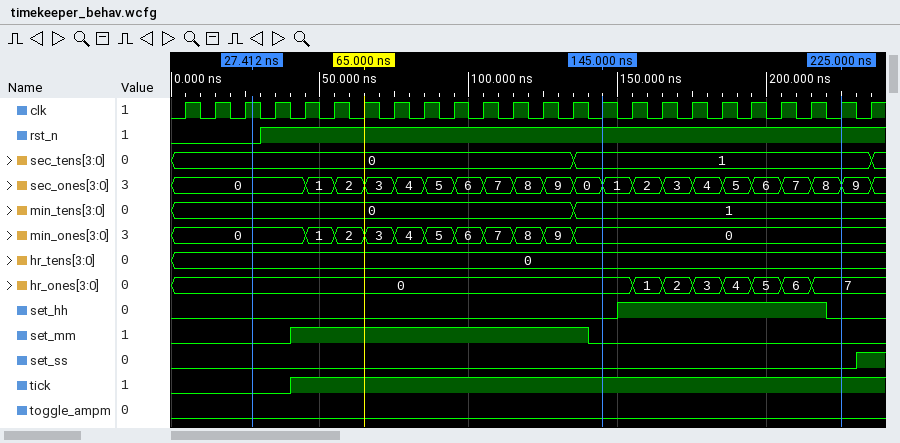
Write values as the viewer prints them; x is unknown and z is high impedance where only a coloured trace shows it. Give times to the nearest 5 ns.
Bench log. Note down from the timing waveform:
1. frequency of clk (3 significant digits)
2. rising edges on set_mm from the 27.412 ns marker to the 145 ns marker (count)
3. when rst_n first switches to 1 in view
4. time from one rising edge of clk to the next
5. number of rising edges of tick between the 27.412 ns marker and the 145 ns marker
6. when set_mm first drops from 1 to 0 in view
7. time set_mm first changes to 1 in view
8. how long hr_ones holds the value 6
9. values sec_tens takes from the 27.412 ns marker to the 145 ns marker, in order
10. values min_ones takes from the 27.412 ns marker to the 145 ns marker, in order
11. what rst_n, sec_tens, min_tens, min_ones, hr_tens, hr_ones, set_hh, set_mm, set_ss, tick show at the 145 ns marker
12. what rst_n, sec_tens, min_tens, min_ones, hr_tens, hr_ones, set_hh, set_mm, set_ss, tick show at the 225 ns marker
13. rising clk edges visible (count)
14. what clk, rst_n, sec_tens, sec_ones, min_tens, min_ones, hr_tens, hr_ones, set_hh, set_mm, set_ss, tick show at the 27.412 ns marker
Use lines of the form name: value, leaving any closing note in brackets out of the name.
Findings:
frequency of clk: 100 MHz
rising edges on set_mm from the 27.412 ns marker to the 145 ns marker: 1
when rst_n first switches to 1 in view: 30 ns
time from one rising edge of clk to the next: 10 ns
number of rising edges of tick between the 27.412 ns marker and the 145 ns marker: 1
when set_mm first drops from 1 to 0 in view: 140 ns
time set_mm first changes to 1 in view: 40 ns
how long hr_ones holds the value 6: 10 ns
values sec_tens takes from the 27.412 ns marker to the 145 ns marker, in order: 0, 1
values min_ones takes from the 27.412 ns marker to the 145 ns marker, in order: 0, 1, 2, 3, 4, 5, 6, 7, 8, 9, 0
what rst_n, sec_tens, min_tens, min_ones, hr_tens, hr_ones, set_hh, set_mm, set_ss, tick show at the 145 ns marker: rst_n=1, sec_tens=1, min_tens=1, min_ones=0, hr_tens=0, hr_ones=0, set_hh=0, set_mm=0, set_ss=0, tick=1
what rst_n, sec_tens, min_tens, min_ones, hr_tens, hr_ones, set_hh, set_mm, set_ss, tick show at the 225 ns marker: rst_n=1, sec_tens=1, min_tens=1, min_ones=0, hr_tens=0, hr_ones=7, set_hh=0, set_mm=0, set_ss=0, tick=1
rising clk edges visible: 24
what clk, rst_n, sec_tens, sec_ones, min_tens, min_ones, hr_tens, hr_ones, set_hh, set_mm, set_ss, tick show at the 27.412 ns marker: clk=1, rst_n=0, sec_tens=0, sec_ones=0, min_tens=0, min_ones=0, hr_tens=0, hr_ones=0, set_hh=0, set_mm=0, set_ss=0, tick=0
